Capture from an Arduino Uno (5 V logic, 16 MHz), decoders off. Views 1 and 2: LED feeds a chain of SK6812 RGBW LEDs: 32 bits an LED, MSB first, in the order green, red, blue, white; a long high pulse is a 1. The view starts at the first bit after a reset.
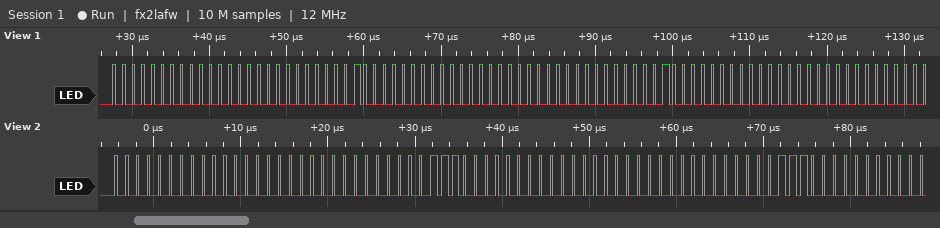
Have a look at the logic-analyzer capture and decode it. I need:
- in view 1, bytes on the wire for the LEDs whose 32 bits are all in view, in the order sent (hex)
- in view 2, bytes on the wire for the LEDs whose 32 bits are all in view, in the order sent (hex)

00 00 00 40 00 00 00 40
00 00 00 07 00 00 00 07
